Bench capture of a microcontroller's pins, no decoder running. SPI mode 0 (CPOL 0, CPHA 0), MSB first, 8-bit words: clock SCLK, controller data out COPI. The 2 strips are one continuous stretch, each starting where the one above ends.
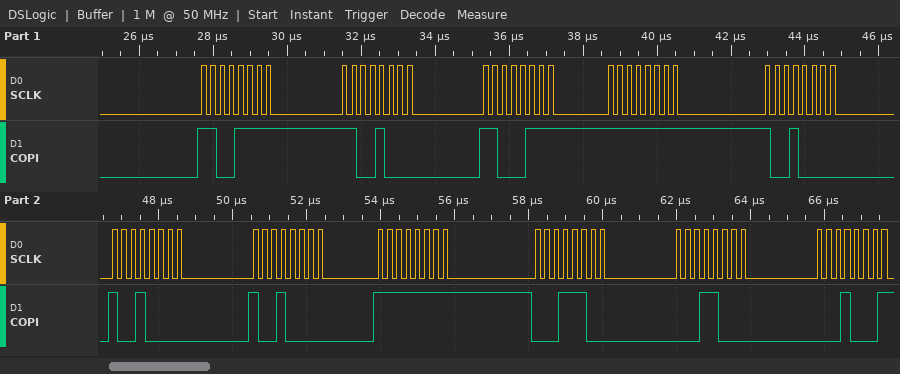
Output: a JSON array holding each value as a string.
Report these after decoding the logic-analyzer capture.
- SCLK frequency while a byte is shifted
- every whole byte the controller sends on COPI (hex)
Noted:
["4 MHz", "CF C8 C7 FF 90 90 90 FF 1C 18 11"]
